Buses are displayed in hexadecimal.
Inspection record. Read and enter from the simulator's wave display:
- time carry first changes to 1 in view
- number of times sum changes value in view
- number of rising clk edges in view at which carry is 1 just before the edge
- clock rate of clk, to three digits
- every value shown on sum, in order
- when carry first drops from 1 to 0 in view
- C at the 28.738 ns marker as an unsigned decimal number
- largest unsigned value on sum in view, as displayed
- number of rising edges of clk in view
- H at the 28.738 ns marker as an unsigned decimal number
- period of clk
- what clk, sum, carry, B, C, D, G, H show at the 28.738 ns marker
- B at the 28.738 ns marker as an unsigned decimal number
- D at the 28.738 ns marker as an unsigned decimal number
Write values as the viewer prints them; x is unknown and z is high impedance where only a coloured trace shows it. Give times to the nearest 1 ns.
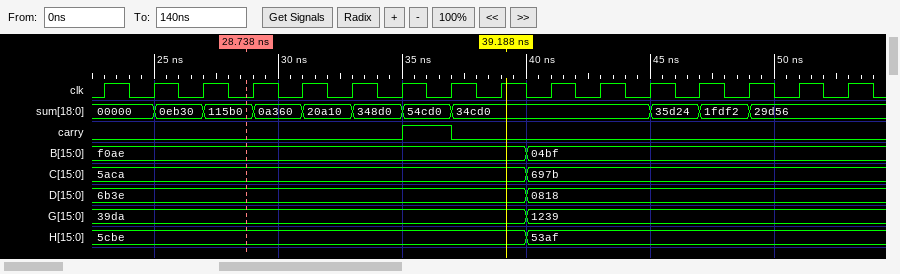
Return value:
35 ns
10
1
500 MHz
00000, 0eb30, 115b0, 0a360, 20a10, 348d0, 54cd0, 34cd0, 35d24, 1fdf2, 29d56
37 ns
23242
54cd0
16
23742
2 ns
clk=0, sum=115b0, carry=0, B=f0ae, C=5aca, D=6b3e, G=39da, H=5cbe
61614
27454
